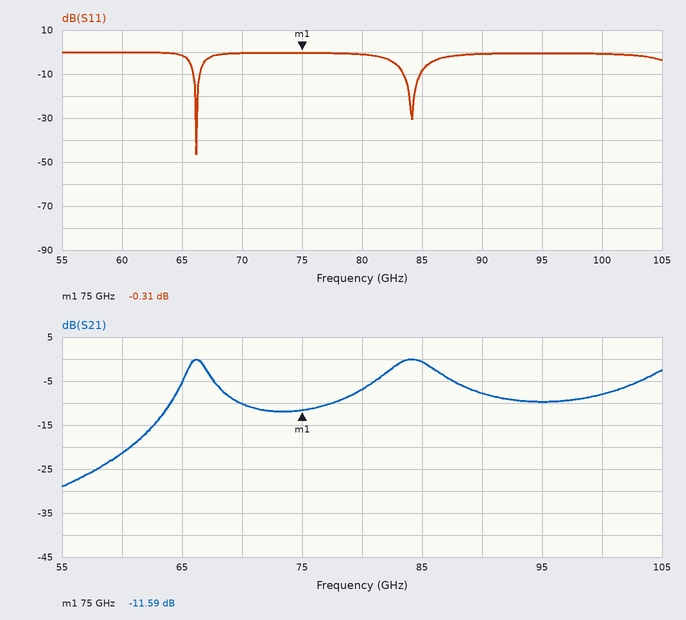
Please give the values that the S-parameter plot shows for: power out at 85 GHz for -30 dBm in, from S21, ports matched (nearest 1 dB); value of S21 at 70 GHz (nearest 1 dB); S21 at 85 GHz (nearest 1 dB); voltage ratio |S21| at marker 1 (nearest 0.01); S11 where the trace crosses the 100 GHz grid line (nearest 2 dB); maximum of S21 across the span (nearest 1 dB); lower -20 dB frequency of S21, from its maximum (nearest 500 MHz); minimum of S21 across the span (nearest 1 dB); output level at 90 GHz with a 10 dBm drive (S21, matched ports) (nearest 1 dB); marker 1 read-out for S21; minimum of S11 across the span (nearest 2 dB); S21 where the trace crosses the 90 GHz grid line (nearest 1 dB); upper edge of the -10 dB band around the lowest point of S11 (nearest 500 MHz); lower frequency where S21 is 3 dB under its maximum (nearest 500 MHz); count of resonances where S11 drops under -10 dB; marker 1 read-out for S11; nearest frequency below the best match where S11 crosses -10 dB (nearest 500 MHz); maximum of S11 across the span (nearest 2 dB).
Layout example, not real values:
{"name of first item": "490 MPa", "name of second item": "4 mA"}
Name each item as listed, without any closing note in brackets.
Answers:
{"power out at 85 GHz for -30 dBm in, from S21, ports matched": "-31 dBm", "value of S21 at 70 GHz": "-10 dB", "S21 at 85 GHz": "-1 dB", "voltage ratio |S21| at marker 1": "0.26", "S11 where the trace crosses the 100 GHz grid line": "0 dB", "maximum of S21 across the span": "0 dB", "lower -20 dB frequency of S21, from its maximum": "60.5 GHz", "minimum of S21 across the span": "-29 dB", "output level at 90 GHz with a 10 dBm drive (S21, matched ports)": "2 dBm", "marker 1 read-out for S21": "-11.59 dB", "minimum of S11 across the span": "-46 dB", "S21 where the trace crosses the 90 GHz grid line": "-8 dB", "upper edge of the -10 dB band around the lowest point of S11": "66.5 GHz", "lower frequency where S21 is 3 dB under its maximum": "65.5 GHz", "count of resonances where S11 drops under -10 dB": "2", "marker 1 read-out for S11": "-0.31 dB", "nearest frequency below the best match where S11 crosses -10 dB": "66.0 GHz", "maximum of S11 across the span": "0 dB"}
